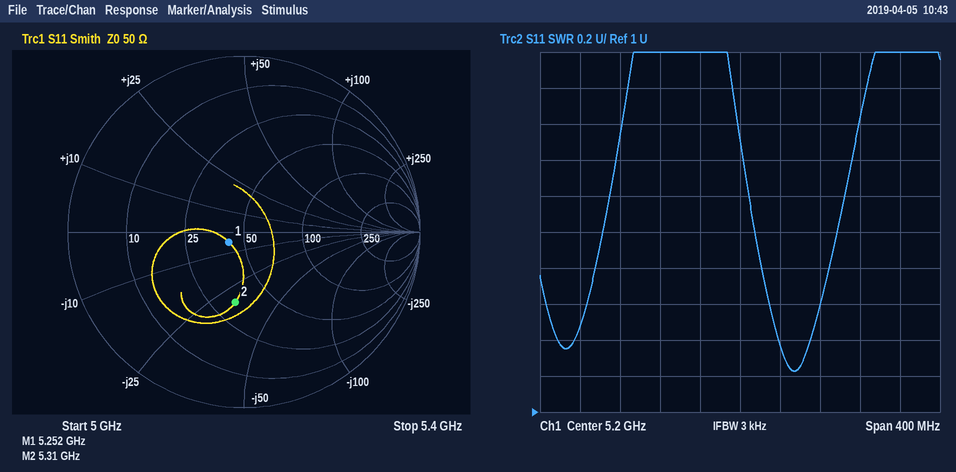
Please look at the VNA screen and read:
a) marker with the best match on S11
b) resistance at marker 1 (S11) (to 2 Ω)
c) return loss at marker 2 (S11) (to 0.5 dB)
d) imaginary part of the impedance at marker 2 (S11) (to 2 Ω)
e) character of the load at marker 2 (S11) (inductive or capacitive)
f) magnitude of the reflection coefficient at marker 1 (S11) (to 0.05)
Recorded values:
marker 1
42 Ω
8.0 dB
-32 Ω
capacitive
0.10
